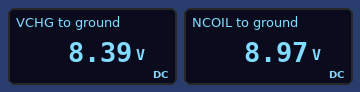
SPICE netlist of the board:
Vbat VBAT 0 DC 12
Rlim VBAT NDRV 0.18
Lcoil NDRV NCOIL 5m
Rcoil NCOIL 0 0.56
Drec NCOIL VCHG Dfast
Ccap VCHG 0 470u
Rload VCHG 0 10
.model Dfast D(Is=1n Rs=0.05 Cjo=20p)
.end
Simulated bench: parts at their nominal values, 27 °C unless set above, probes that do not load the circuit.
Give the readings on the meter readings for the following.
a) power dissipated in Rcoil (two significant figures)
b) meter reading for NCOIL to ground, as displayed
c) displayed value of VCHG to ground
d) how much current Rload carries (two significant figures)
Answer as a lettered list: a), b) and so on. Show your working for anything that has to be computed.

a) (8.97 V)^2 / 560 mΩ = 140 W
b) 8.97 V
c) 8.39 V
d) (8.39 V) / 10 Ω = 840 mA
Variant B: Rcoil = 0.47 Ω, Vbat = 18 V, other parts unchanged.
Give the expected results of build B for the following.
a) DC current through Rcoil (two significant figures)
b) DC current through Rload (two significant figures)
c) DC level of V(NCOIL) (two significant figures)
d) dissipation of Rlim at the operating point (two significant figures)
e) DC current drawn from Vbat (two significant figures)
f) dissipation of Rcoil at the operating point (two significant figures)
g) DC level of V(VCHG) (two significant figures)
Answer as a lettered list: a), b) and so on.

a) 27 A
b) 1.2 A
c) 13 V
d) 150 W
e) 29 A
f) 350 W
g) 12 V
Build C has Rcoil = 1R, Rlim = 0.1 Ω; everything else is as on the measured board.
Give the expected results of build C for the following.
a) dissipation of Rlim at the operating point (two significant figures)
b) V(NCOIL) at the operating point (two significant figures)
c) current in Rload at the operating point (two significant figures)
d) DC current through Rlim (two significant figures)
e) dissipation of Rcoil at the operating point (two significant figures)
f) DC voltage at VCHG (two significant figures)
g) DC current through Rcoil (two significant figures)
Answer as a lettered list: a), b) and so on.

a) 14 W
b) 11 V
c) 1.0 A
d) 12 A
e) 120 W
f) 10 V
g) 11 A
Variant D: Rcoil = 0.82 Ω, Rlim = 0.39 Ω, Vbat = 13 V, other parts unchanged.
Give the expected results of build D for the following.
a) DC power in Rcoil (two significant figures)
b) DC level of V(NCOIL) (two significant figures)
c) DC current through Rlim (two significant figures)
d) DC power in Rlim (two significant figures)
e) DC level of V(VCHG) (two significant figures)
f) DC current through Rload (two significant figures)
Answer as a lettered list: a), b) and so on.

a) 90 W
b) 8.6 V
c) 11 A
d) 50 W
e) 8.0 V
f) 800 mA
